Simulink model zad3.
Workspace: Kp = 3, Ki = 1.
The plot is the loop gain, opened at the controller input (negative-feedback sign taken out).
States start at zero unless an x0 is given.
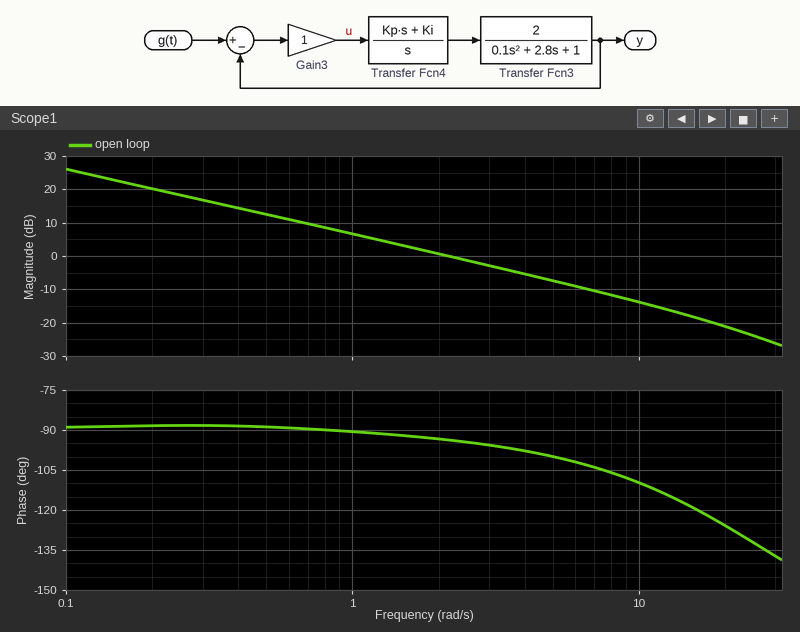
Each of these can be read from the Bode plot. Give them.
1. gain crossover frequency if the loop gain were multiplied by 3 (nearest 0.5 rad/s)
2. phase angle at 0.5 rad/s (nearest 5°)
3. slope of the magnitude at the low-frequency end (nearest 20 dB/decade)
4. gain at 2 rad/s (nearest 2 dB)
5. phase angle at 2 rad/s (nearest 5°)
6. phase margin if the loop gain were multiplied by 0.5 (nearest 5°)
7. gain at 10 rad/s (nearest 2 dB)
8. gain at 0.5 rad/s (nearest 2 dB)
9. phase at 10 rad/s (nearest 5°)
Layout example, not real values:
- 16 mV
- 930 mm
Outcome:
- 6.5 rad/s
- -90°
- -20 dB/decade
- 0 dB
- -95°
- 90°
- -14 dB
- 12 dB
- -110°
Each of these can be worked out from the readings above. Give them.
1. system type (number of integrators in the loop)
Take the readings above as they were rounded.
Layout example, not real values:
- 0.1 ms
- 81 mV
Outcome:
- 1
